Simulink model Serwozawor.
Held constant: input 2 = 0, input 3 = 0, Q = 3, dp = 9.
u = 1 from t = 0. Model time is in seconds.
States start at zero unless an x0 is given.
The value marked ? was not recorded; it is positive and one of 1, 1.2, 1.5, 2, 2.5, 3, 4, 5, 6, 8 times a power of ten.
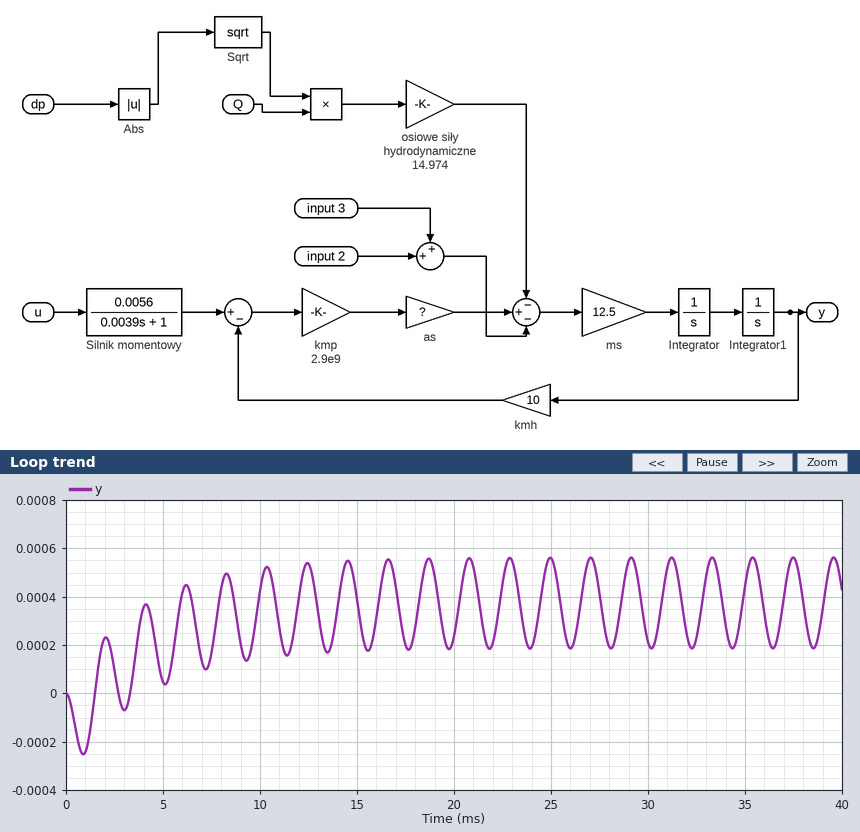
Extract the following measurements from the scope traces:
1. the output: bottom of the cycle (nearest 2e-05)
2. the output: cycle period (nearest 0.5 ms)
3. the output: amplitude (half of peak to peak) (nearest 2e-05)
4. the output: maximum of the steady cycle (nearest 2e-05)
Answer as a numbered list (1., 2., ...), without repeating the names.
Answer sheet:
1. 0.00018
2. 2.0 ms
3. 0.00018
4. 0.00056
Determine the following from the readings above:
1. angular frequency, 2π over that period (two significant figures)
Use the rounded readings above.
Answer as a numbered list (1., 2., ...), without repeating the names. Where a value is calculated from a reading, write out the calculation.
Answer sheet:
1. 2π / 2 = 3.1 rad/ms
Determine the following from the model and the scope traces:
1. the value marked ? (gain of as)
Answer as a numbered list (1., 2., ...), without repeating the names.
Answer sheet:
1. 2.5e-05
